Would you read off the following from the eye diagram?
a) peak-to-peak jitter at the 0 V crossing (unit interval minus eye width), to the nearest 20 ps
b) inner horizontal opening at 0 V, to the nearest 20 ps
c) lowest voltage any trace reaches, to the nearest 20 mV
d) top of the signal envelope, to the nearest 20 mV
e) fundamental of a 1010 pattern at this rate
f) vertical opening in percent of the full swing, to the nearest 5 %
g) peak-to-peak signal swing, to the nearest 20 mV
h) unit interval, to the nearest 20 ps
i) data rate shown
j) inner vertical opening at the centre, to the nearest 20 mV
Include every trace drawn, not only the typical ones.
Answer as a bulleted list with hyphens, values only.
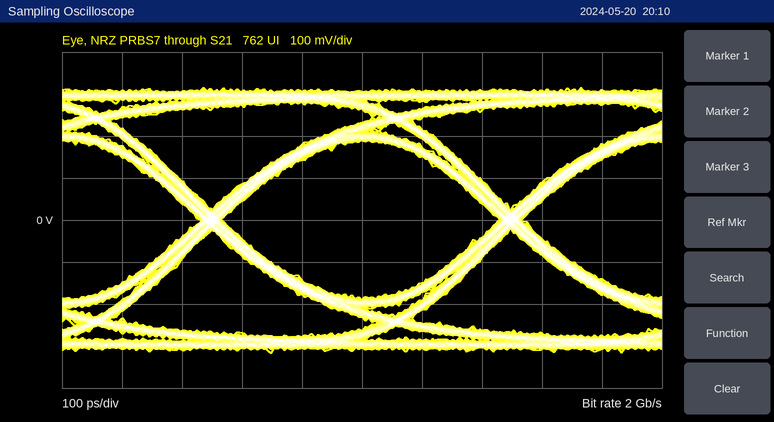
- 40 ps
- 460 ps
- -320 mV
- 320 mV
- 1 GHz
- 60 %
- 640 mV
- 500 ps
- 2 Gb/s
- 380 mV
